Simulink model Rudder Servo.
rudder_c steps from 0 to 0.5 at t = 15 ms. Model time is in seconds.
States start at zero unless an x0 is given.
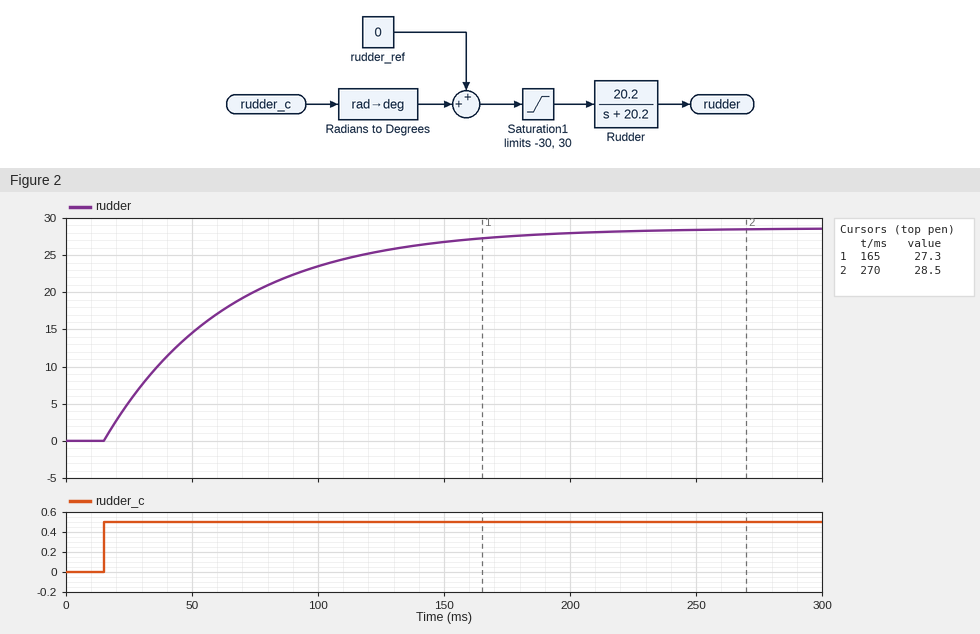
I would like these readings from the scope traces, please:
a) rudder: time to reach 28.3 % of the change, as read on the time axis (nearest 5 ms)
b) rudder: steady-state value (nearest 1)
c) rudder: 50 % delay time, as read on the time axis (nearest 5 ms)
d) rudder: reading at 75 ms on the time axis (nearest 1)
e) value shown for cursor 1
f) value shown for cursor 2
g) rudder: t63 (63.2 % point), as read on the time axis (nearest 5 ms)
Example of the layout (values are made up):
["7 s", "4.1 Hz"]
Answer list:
["30 ms", "29", "50 ms", "20", "27.3", "28.5", "65 ms"]
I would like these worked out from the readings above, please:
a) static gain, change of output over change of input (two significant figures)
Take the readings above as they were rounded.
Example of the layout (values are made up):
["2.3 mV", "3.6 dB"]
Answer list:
["58"]
